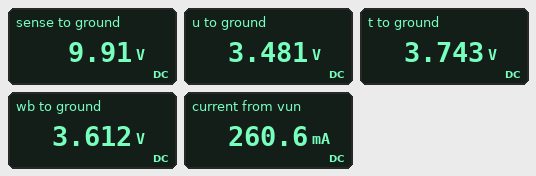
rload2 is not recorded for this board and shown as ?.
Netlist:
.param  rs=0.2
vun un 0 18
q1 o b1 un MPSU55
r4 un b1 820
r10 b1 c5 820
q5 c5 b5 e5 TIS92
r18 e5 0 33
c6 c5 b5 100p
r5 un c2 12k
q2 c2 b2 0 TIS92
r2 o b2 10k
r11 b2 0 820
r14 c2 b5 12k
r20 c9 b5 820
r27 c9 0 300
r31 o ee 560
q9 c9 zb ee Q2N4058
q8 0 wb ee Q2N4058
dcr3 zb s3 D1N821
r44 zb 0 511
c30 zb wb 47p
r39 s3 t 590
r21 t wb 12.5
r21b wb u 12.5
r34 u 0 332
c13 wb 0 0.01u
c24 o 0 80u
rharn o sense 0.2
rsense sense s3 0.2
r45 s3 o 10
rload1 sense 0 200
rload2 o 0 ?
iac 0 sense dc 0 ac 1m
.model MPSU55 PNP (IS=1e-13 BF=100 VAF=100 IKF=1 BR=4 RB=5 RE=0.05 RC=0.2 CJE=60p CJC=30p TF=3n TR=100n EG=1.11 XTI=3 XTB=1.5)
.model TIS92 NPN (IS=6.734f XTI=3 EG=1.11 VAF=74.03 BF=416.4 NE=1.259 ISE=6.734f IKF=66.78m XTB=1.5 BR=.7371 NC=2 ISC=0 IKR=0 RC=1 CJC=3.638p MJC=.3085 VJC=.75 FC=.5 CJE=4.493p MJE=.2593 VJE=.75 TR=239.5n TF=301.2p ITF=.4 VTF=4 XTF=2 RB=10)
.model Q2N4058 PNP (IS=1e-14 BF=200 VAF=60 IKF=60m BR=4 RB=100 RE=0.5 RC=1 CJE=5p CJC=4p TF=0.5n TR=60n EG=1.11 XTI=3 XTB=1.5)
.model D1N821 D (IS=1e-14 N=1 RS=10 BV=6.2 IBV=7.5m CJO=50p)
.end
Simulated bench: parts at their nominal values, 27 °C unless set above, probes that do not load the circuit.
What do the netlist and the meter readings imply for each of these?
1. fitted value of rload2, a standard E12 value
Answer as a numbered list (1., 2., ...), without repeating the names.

1. 56 Ω
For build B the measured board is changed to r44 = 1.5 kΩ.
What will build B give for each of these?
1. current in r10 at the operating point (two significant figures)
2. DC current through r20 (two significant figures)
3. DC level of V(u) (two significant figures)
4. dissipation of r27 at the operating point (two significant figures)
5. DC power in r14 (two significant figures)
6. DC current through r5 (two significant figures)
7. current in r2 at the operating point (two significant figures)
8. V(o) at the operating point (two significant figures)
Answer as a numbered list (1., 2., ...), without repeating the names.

1. 3.8 mA
2. 82 µA
3. 3.4 V
4. 2.6 mW
5. 44 µW
6. 1.5 mA
7. 910 µA
8. 9.8 V
